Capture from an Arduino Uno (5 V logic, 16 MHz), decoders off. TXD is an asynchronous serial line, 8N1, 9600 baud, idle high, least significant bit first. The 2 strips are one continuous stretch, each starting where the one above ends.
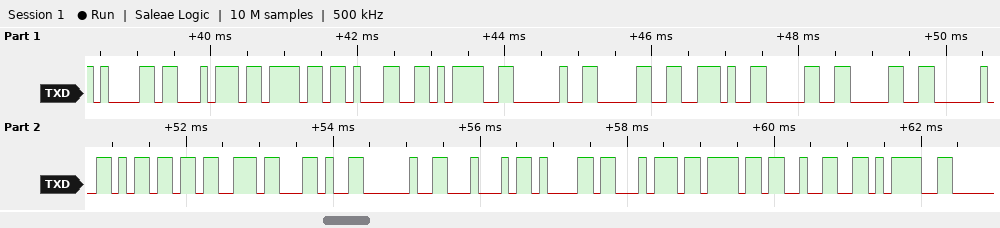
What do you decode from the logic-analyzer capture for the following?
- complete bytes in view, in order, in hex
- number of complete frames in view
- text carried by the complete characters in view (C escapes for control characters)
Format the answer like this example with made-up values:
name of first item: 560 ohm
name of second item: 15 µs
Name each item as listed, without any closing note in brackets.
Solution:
complete bytes in view, in order, in hex: 61 74 6F 31 3D 20 30 2E 30 30 20 6D 73 2C 20 44 61 74 6F 32 3D
number of complete frames in view: 21
text carried by the complete characters in view: "ato1= 0.00 ms, Dato2="
